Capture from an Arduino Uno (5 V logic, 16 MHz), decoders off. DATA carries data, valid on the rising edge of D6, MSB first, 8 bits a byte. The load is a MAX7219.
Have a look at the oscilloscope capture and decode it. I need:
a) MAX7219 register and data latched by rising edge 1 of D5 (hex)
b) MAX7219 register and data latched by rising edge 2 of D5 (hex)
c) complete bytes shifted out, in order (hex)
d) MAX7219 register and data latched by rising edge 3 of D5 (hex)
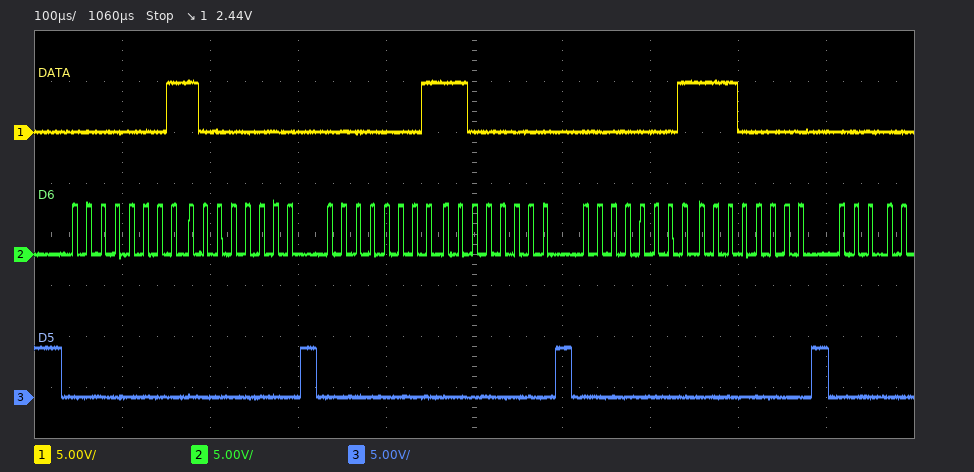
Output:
register 0x1, data 0x80
register 0x1, data 0xC0
01 80 01 C0 01 E0
register 0x1, data 0xE0
